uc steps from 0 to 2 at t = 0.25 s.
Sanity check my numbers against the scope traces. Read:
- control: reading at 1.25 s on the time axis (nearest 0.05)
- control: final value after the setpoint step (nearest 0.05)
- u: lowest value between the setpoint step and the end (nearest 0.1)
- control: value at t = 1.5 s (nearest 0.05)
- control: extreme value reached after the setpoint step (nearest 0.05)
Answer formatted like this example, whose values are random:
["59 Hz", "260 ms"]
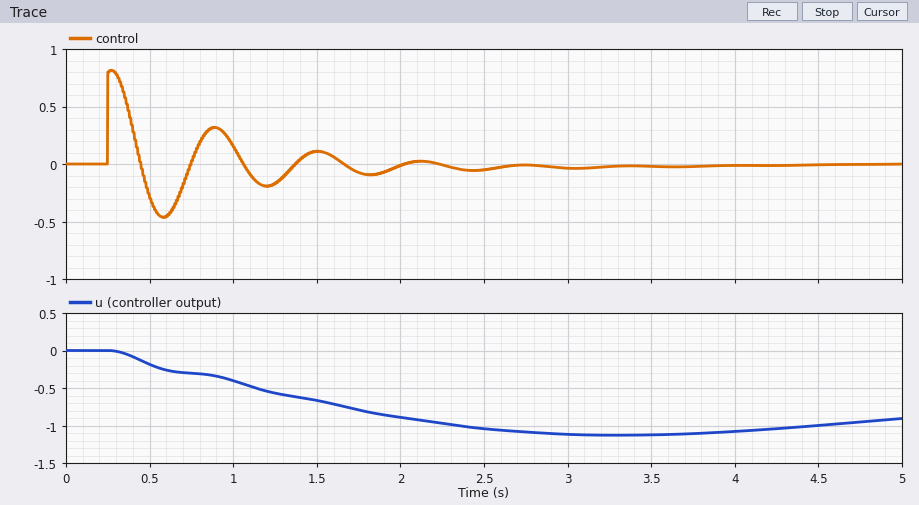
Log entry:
["-0.15", "0.00", "-1.1", "0.10", "0.80"]
